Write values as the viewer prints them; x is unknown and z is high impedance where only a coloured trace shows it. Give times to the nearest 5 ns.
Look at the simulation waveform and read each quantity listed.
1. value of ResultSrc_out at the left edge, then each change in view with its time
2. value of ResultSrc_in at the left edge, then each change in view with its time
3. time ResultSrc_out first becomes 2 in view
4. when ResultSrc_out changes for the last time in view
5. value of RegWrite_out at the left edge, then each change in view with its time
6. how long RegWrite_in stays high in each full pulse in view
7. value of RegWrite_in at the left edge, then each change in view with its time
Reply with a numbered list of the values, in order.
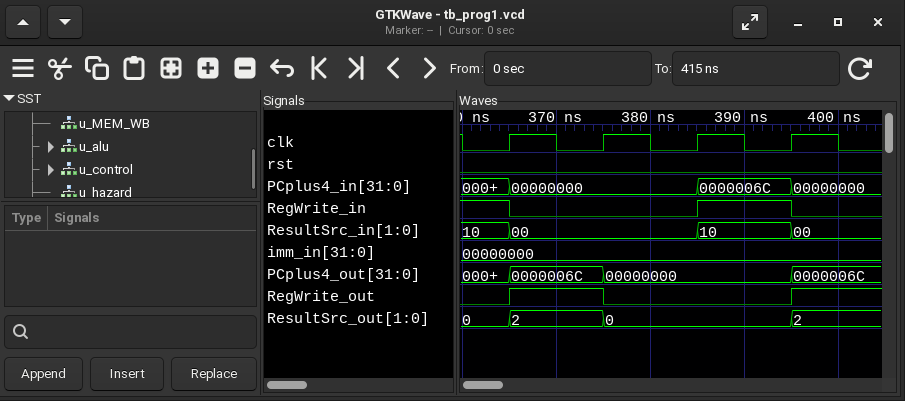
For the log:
1. 0, 2 at 365 ns, 0 at 375 ns, 2 at 395 ns
2. 10, 00 at 365 ns, 10 at 385 ns, 00 at 395 ns
3. 365 ns
4. 395 ns
5. 0, 1 at 365 ns, 0 at 375 ns, 1 at 395 ns
6. 10 ns
7. 1, 0 at 365 ns, 1 at 385 ns, 0 at 395 ns
